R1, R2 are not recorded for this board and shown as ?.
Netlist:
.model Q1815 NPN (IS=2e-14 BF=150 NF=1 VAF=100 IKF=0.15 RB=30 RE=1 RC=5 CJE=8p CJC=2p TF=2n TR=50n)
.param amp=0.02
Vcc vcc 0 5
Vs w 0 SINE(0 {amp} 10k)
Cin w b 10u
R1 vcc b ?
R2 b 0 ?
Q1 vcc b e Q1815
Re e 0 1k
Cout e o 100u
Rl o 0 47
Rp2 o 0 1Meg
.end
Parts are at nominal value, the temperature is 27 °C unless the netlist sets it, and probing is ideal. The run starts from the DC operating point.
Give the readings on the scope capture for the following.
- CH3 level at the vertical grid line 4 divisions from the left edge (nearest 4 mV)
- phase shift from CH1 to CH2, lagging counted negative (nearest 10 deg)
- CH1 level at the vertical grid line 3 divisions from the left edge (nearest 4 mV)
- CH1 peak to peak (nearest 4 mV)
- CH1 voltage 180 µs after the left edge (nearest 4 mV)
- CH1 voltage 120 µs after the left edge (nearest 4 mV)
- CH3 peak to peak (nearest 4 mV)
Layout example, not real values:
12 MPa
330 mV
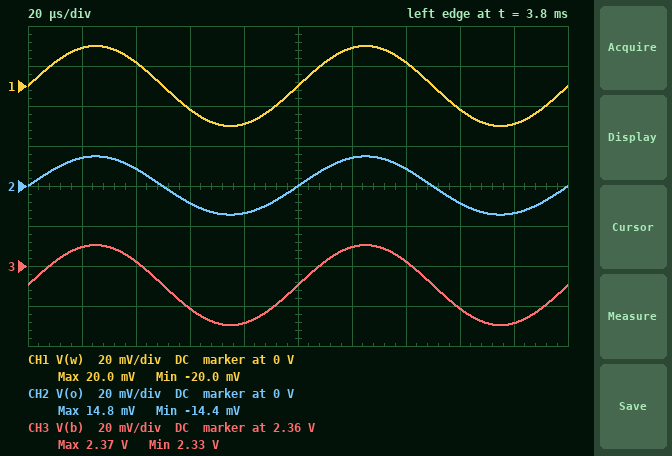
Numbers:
2.332 V
0 deg
-12 mV
40 mV
-20 mV
20 mV
40 mV
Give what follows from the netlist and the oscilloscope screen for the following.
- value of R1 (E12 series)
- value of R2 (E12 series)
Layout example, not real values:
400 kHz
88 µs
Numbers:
27 kΩ
27 kΩ
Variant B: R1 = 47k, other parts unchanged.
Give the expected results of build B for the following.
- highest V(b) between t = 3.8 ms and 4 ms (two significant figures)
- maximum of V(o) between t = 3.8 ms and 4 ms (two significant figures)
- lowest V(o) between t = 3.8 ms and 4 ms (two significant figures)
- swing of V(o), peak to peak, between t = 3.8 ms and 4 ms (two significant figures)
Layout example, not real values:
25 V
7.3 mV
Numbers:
1.7 V
13 mV
-12 mV
25 mV
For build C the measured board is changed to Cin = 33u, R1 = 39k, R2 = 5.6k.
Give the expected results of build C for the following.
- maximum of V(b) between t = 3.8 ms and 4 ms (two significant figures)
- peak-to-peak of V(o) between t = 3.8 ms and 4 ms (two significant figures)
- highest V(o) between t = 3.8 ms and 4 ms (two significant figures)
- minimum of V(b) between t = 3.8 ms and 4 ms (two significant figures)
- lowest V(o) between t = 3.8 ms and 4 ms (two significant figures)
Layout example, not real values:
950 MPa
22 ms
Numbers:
650 mV
4.0 mV
2.6 mV
610 mV
-1.4 mV
